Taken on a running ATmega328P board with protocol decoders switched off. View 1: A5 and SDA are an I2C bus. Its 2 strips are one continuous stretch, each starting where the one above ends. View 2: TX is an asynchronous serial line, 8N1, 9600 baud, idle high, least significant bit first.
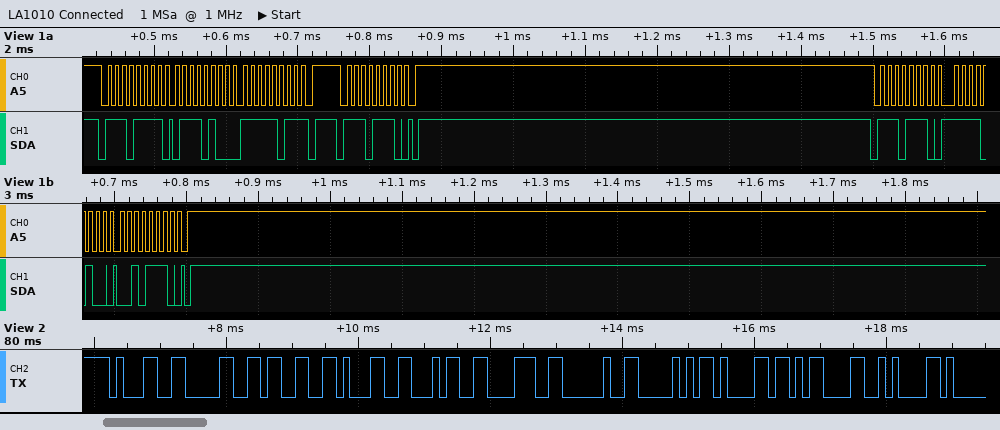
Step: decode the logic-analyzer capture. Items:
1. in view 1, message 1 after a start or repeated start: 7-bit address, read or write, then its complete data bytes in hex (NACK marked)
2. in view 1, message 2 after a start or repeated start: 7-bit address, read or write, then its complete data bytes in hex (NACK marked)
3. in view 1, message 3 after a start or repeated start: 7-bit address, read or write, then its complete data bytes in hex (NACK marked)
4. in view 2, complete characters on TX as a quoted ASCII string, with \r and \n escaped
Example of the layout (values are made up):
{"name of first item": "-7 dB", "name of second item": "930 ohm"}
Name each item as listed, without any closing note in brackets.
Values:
{"in view 1, message 1 after a start or repeated start: 7-bit address, read or write, then its complete data bytes in hex": "0x77 read: 74 FB NACK", "in view 1, message 2 after a start or repeated start: 7-bit address, read or write, then its complete data bytes in hex": "0x77 write", "in view 1, message 3 after a start or repeated start: 7-bit address, read or write, then its complete data bytes in hex": "0x77 write: F4 2E", "in view 2, complete characters on TX as a quoted ASCII string, with \\r and \\n escaped": "\"103148 Pa\\r\\n\""}
